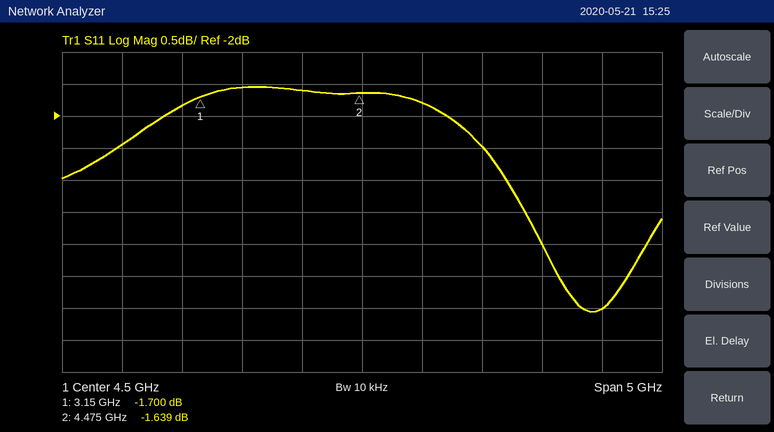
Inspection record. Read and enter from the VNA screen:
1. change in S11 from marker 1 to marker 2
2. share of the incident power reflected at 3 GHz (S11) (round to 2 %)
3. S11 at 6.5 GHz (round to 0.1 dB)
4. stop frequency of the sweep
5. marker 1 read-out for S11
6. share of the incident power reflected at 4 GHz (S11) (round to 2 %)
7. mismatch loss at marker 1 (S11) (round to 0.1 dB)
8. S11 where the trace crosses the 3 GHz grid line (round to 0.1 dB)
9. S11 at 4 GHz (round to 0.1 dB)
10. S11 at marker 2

0.061 dB
66 %
-5.0 dB
7 GHz
-1.700 dB
70 %
4.9 dB
-1.8 dB
-1.6 dB
-1.639 dB
